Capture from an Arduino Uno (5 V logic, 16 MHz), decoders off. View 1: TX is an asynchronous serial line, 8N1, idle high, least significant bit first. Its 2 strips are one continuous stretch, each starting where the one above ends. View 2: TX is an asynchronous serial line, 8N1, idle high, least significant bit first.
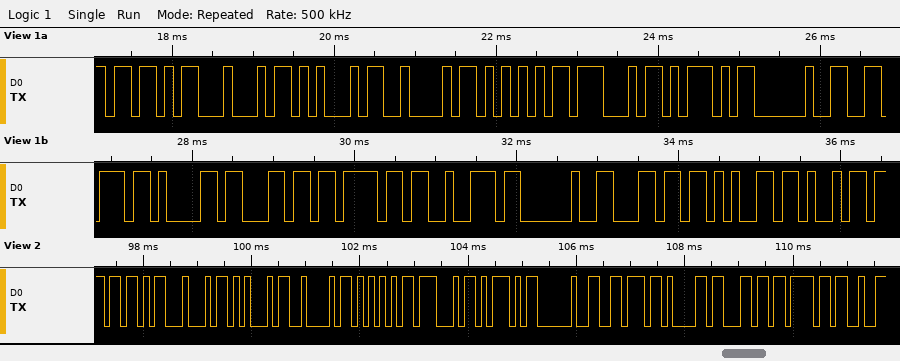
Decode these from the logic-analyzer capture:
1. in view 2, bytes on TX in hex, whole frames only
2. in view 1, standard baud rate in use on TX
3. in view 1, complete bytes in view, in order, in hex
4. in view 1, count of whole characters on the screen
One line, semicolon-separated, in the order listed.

5B 44 45 42 55 47 5D 20 76 61 6C 6F; 9600 baud; 5B 44 45 42 55 47 5D 20 76 61 6C 6F 72 20 6C 65 69; 17
